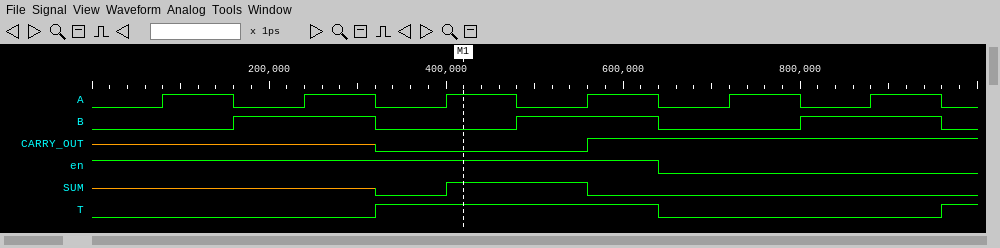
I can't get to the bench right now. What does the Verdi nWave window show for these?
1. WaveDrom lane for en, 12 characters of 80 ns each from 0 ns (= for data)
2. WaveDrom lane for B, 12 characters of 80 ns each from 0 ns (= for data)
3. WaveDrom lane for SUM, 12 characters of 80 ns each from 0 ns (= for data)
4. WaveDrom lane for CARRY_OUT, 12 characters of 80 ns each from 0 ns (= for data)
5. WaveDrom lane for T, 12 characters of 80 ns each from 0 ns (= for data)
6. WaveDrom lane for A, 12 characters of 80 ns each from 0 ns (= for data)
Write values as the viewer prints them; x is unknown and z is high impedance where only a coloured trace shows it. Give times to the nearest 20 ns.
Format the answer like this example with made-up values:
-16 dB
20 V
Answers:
{name: 'en', wave: '1.......0...'}
{name: 'B', wave: '0.1.0.1.0.1.'}
{name: 'SUM', wave: 'z...01.0....'}
{name: 'CARRY_OUT', wave: 'z...0..1....'}
{name: 'T', wave: '0...1...0...'}
{name: 'A', wave: '010101010101'}
